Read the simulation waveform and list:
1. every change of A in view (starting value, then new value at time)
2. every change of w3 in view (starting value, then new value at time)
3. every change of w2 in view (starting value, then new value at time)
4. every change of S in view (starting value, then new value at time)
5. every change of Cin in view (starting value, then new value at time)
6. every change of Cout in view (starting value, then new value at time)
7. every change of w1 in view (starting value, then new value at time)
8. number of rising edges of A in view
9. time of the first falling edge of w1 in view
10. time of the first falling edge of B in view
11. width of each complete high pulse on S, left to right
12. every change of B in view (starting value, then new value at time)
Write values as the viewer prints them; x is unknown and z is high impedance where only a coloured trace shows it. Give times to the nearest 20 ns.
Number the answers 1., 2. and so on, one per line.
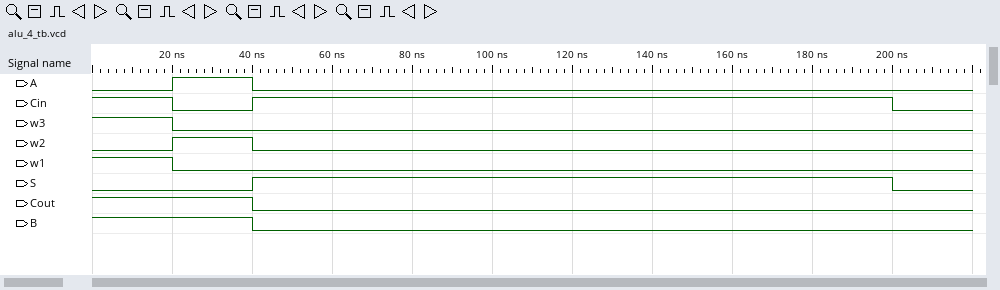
1. 0, 1 at 20 ns, 0 at 40 ns
2. 1, 0 at 20 ns
3. 0, 1 at 20 ns, 0 at 40 ns
4. 0, 1 at 40 ns, 0 at 200 ns
5. 1, 0 at 20 ns, 1 at 40 ns, 0 at 200 ns
6. 1, 0 at 40 ns
7. 1, 0 at 20 ns
8. 1
9. 20 ns
10. 40 ns
11. 160 ns
12. 1, 0 at 40 ns
